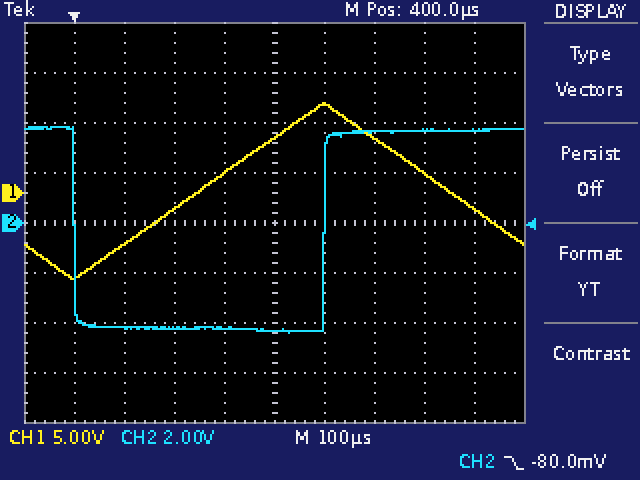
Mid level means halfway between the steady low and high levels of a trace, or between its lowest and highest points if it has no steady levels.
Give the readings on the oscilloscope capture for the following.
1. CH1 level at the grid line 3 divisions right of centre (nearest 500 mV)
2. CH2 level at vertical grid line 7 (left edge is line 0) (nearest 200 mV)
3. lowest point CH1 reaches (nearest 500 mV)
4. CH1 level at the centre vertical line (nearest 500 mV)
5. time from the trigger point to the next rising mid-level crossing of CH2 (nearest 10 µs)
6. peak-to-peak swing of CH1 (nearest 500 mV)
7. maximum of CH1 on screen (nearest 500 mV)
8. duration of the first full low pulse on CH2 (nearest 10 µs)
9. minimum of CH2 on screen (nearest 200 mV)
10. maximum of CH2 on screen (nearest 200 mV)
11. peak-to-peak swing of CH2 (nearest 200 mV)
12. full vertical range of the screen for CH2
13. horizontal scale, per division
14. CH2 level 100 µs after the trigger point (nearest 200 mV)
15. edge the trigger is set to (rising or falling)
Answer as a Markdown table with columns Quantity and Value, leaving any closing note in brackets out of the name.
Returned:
| Quantity | Value |
|---|---|
| CH1 level at the grid line 3 divisions right of centre | 2.0 V |
| CH2 level at vertical grid line 7 (left edge is line 0) | 3.6 V |
| lowest point CH1 reaches | -8.5 V |
| CH1 level at the centre vertical line | 5.5 V |
| time from the trigger point to the next rising mid-level crossing of CH2 | 500 µs |
| peak-to-peak swing of CH1 | 17.5 V |
| maximum of CH1 on screen | 9.0 V |
| duration of the first full low pulse on CH2 | 500 µs |
| minimum of CH2 on screen | -4.4 V |
| maximum of CH2 on screen | 3.8 V |
| peak-to-peak swing of CH2 | 8.2 V |
| full vertical range of the screen for CH2 | 16 V |
| horizontal scale, per division | 100 µs |
| CH2 level 100 µs after the trigger point | -4.2 V |
| edge the trigger is set to | falling |
